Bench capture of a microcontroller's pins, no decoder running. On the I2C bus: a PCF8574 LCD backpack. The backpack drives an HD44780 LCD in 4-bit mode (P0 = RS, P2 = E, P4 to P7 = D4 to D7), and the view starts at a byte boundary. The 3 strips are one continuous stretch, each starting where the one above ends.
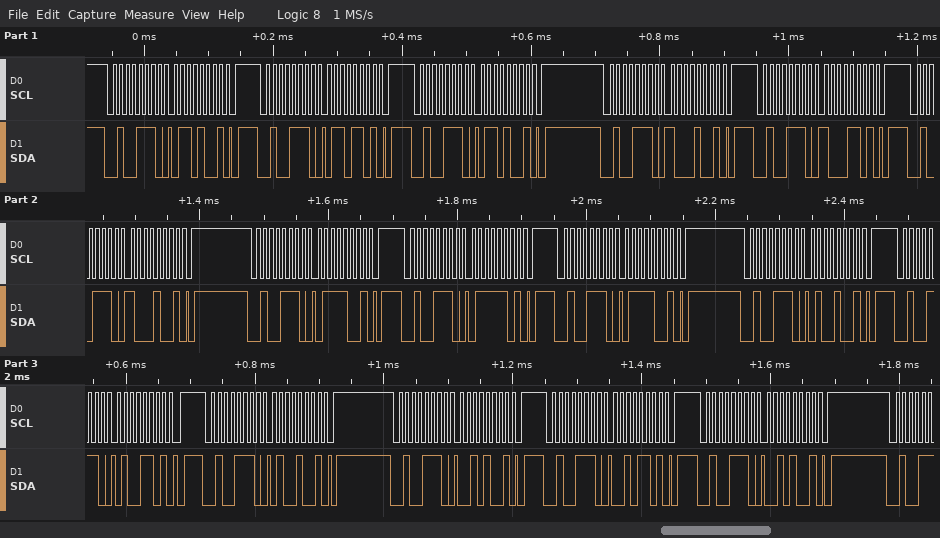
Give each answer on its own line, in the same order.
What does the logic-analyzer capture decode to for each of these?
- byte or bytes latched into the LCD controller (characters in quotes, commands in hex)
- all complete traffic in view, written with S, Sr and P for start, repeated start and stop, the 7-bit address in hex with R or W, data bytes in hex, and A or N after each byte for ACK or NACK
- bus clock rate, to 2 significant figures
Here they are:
'h' 't'
S 27W A 69 A P S 27W A 6D A P S 27W A 69 A P S 27W A 89 A P S 27W A 8D A P S 27W A 89 A P S 27W A 79 A P S 27W A 7D A P S 27W A 79 A P S 27W A 49 A P S 27W A 4D A P S 27W A 49 A P S 27W A 29 A P S 27W A 2D A P S 27W A 29 A P
100 kHz
